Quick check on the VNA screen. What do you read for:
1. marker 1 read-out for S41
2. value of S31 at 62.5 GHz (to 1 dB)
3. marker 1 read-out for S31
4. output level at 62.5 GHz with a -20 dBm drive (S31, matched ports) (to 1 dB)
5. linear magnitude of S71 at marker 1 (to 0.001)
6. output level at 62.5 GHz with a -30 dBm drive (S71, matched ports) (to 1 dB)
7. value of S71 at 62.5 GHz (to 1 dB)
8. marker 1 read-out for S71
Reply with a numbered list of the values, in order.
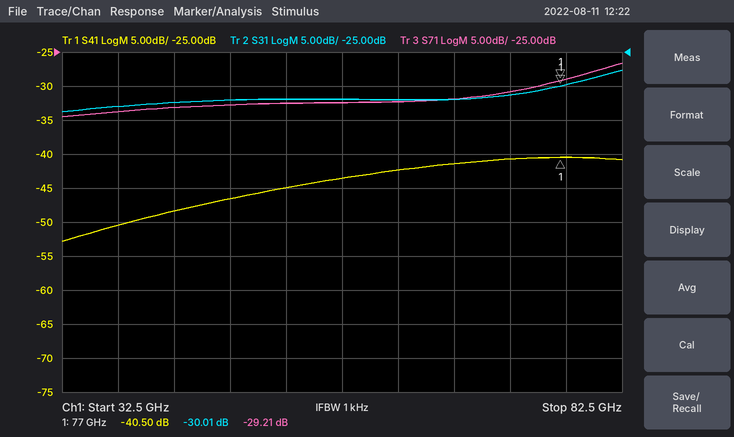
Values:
1. -40.50 dB
2. -32 dB
3. -30.01 dB
4. -52 dBm
5. 0.035
6. -62 dBm
7. -32 dB
8. -29.21 dB
